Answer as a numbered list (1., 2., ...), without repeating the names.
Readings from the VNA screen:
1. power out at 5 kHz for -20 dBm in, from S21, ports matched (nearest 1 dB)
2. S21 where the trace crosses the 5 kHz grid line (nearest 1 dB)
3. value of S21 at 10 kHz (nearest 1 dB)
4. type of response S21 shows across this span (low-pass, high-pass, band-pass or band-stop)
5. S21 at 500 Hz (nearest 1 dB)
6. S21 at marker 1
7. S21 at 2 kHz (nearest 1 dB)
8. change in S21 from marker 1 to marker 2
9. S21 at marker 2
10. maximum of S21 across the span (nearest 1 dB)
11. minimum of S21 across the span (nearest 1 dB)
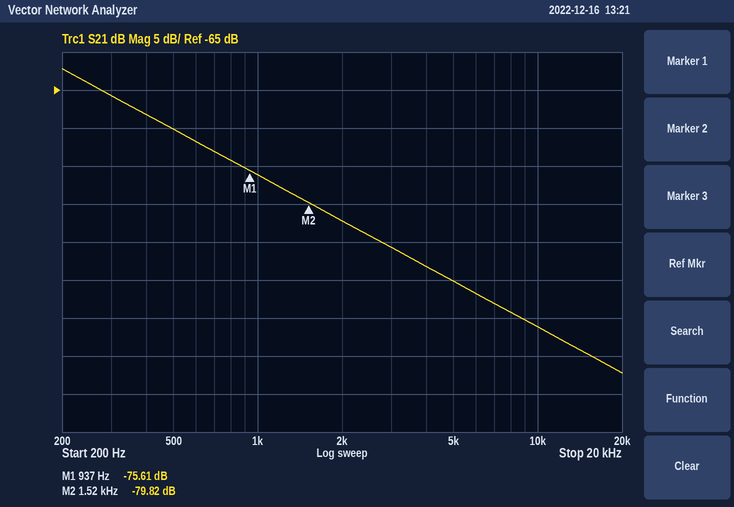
1. -110 dBm
2. -90 dB
3. -96 dB
4. low-pass
5. -70 dB
6. -75.61 dB
7. -82 dB
8. -4.21 dB
9. -79.82 dB
10. -62 dB
11. -102 dB
